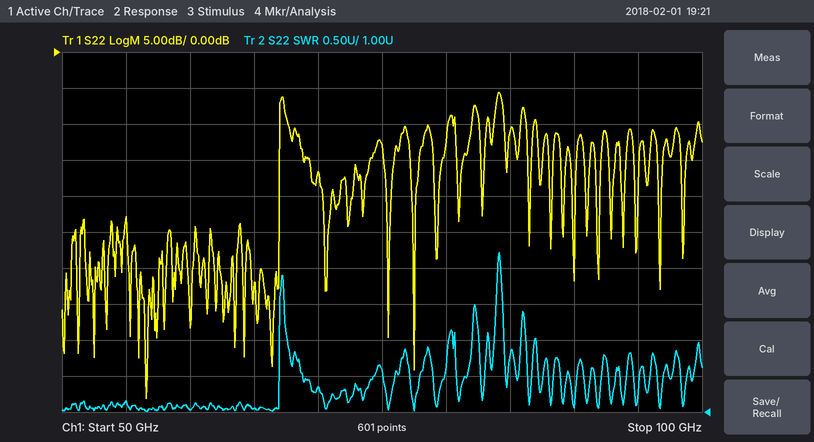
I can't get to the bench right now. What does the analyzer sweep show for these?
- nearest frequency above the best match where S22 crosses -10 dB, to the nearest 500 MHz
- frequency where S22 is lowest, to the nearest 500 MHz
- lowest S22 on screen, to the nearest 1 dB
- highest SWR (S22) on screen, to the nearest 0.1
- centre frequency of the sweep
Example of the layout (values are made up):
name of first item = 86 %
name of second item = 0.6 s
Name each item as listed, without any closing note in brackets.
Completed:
nearest frequency above the best match where S22 crosses -10 dB, to the nearest 500 MHz = 67.0 GHz
frequency where S22 is lowest, to the nearest 500 MHz = 56.5 GHz
lowest S22 on screen, to the nearest 1 dB = -48 dB
highest SWR (S22) on screen, to the nearest 0.1 = 3.2
centre frequency of the sweep = 75 GHz
